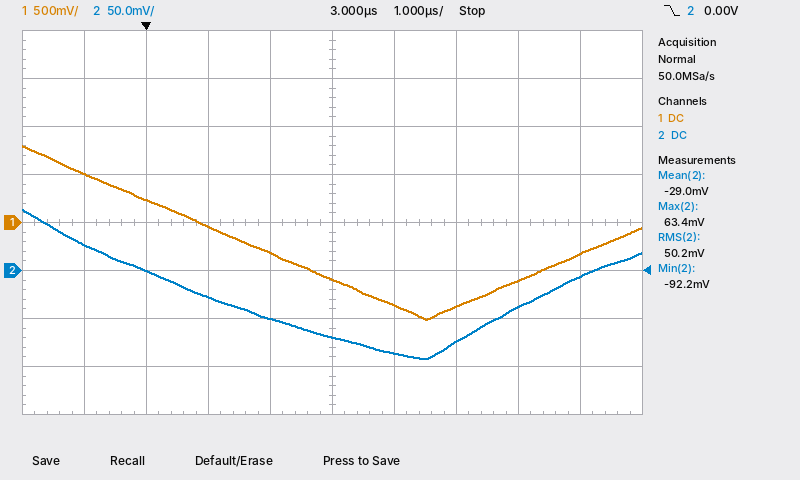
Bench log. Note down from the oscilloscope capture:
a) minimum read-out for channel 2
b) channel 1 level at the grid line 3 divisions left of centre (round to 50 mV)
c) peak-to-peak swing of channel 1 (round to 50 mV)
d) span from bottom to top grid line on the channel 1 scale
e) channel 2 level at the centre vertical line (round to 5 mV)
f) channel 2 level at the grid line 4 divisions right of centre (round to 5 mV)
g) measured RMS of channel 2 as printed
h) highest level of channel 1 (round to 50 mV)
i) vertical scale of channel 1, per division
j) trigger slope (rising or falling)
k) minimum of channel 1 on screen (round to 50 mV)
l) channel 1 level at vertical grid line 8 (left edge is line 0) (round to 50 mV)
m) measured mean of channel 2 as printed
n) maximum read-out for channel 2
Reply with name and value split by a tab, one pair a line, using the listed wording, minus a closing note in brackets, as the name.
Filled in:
minimum read-out for channel 2	-92.2 mV
channel 1 level at the grid line 3 divisions left of centre	250 mV
peak-to-peak swing of channel 1	1.80 V
span from bottom to top grid line on the channel 1 scale	4 V
channel 2 level at the centre vertical line	-70 mV
channel 2 level at the grid line 4 divisions right of centre	-5 mV
measured RMS of channel 2 as printed	50.2 mV
highest level of channel 1	800 mV
vertical scale of channel 1, per division	500 mV
trigger slope	falling
minimum of channel 1 on screen	-1.00 V
channel 1 level at vertical grid line 8 (left edge is line 0)	-600 mV
measured mean of channel 2 as printed	-29.0 mV
maximum read-out for channel 2	63.4 mV
